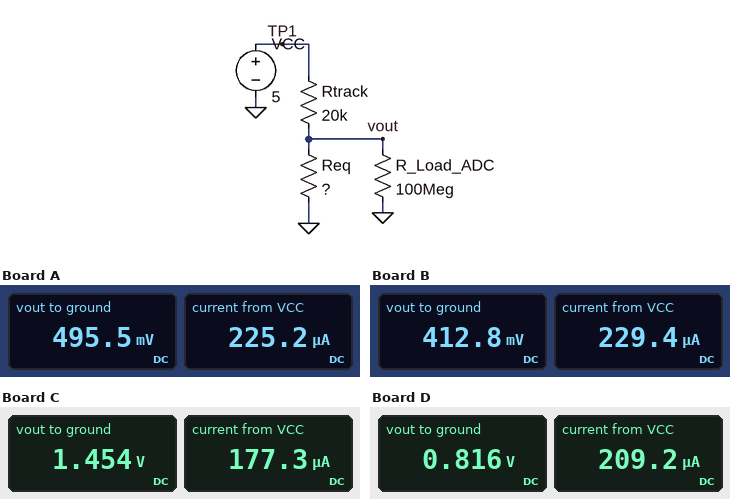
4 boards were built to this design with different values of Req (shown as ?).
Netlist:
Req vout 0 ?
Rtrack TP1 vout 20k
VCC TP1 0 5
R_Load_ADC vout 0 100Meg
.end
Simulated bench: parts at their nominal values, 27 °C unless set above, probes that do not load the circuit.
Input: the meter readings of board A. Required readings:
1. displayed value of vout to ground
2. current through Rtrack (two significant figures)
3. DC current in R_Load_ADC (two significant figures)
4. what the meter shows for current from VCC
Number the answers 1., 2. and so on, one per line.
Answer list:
1. 495.5 mV
2. 230 µA
3. 5.0 nA
4. 225.2 µA
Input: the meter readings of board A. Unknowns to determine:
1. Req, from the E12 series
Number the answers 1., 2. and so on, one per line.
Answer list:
1. 2.2 kΩ
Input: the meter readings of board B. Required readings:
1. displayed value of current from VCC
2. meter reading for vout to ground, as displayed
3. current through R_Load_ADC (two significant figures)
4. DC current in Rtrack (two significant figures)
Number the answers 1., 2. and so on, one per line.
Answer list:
1. 229.4 µA
2. 412.8 mV
3. 4.1 nA
4. 230 µA
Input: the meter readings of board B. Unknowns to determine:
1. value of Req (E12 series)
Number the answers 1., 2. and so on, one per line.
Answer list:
1. 1.8 kΩ
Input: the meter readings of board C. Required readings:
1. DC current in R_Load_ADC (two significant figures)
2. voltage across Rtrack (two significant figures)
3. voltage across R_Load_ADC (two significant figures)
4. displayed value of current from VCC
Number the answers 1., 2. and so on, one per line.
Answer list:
1. 15 nA
2. 3.5 V
3. 1.5 V
4. 177.3 µA
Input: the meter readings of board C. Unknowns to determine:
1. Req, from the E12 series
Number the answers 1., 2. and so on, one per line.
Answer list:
1. 8.2 kΩ
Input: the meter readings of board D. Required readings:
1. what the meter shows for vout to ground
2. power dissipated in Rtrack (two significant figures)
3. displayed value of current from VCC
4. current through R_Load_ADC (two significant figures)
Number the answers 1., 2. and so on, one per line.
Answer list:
1. 0.816 V
2. 880 µW
3. 209.2 µA
4. 8.2 nA
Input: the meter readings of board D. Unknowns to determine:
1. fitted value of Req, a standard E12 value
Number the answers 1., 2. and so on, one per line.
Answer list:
1. 3.9 kΩ
